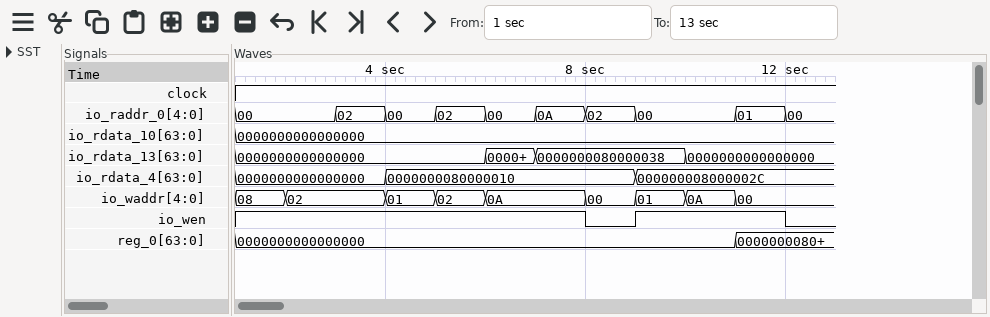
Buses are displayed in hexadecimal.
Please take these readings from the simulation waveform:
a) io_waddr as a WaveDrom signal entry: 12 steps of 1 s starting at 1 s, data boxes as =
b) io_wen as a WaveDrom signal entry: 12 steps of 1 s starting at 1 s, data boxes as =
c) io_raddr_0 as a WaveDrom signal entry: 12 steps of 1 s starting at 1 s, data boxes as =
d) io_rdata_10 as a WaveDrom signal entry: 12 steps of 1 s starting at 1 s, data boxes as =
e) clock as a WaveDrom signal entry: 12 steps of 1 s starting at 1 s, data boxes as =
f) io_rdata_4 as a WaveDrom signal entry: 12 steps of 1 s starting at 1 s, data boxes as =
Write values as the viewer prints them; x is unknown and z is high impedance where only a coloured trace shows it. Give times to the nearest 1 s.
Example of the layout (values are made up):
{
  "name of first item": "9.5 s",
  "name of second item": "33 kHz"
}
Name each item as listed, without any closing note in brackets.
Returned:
{
  "io_waddr as a WaveDrom signal entry: 12 steps of 1 s starting at 1 s, data boxes as =": "{name: 'io_waddr', wave: '==.===.====.', data: '08 02 01 02 0A 00 01 0A 00'}",
  "io_wen as a WaveDrom signal entry: 12 steps of 1 s starting at 1 s, data boxes as =": "{name: 'io_wen', wave: '1......01..0'}",
  "io_raddr_0 as a WaveDrom signal entry: 12 steps of 1 s starting at 1 s, data boxes as =": "{name: 'io_raddr_0', wave: '=.=======.==', data: '00 02 00 02 00 0A 02 00 01 00'}",
  "io_rdata_10 as a WaveDrom signal entry: 12 steps of 1 s starting at 1 s, data boxes as =": "{name: 'io_rdata_10', wave: '=...........', data: '0000000000000000'}",
  "clock as a WaveDrom signal entry: 12 steps of 1 s starting at 1 s, data boxes as =": "{name: 'clock', wave: '1...........'}",
  "io_rdata_4 as a WaveDrom signal entry: 12 steps of 1 s starting at 1 s, data boxes as =": "{name: 'io_rdata_4', wave: '=..=....=...', data: '0000000000000000 0000000080000010 000000008000002C'}"
}
